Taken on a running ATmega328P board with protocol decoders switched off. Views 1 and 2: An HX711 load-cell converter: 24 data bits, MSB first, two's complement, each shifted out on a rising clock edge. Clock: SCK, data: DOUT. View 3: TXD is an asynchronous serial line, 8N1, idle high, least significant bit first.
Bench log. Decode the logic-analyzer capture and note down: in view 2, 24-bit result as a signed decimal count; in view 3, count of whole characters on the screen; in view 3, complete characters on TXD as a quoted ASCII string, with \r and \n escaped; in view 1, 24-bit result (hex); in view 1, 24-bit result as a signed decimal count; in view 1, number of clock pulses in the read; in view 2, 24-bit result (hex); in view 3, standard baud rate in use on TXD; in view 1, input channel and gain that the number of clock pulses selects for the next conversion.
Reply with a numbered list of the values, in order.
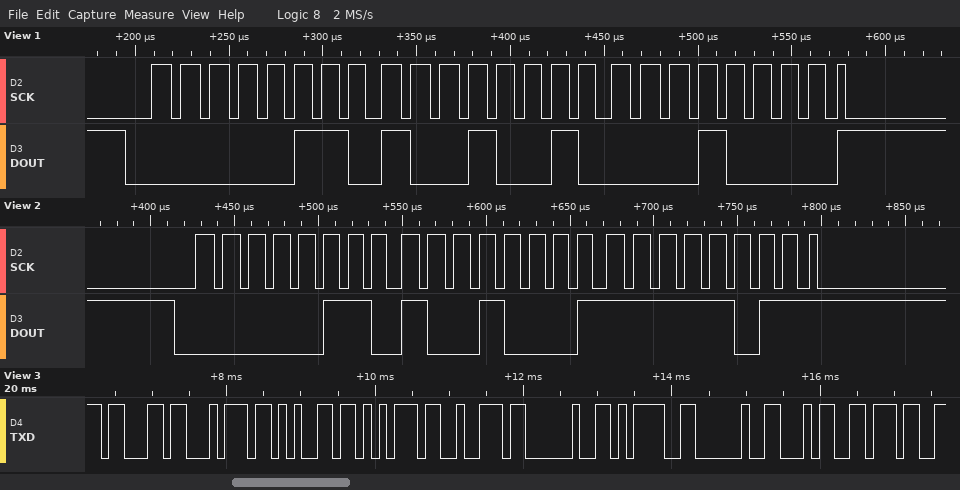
1. 430587
2. 10
3. "cteur = 47"
4. 0x069210
5. 430608
6. 25
7. 0x0691FB
8. 9600 baud
9. channel A, gain 128
